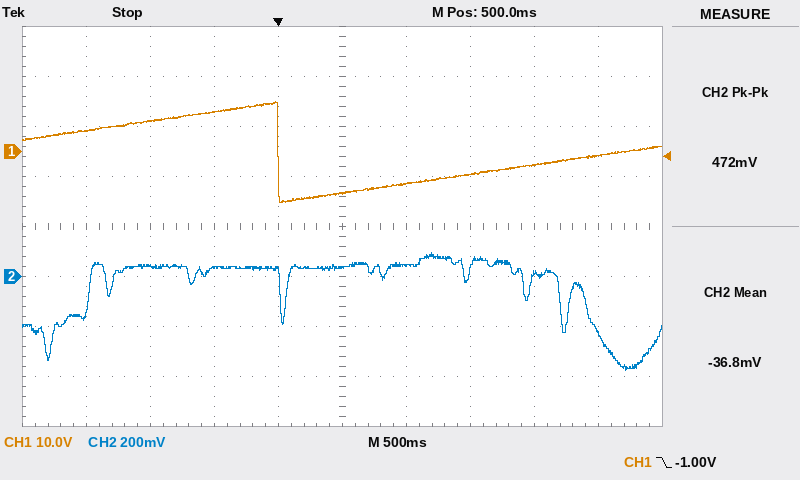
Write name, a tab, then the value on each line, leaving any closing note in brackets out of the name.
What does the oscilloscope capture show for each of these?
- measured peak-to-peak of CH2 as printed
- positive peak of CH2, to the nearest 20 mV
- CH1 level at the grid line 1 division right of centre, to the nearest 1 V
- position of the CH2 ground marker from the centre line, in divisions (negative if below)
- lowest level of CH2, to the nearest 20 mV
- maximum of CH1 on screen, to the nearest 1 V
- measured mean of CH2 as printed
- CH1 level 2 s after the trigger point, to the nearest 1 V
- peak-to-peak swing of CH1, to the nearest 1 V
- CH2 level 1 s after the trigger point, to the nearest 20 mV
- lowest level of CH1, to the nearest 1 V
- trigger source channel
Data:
measured peak-to-peak of CH2 as printed	472 mV
positive peak of CH2, to the nearest 20 mV	100 mV
CH1 level at the grid line 1 division right of centre, to the nearest 1 V	-6 V
position of the CH2 ground marker from the centre line, in divisions	-1.0 div
lowest level of CH2, to the nearest 20 mV	-380 mV
maximum of CH1 on screen, to the nearest 1 V	10 V
measured mean of CH2 as printed	-36.8 mV
CH1 level 2 s after the trigger point, to the nearest 1 V	-3 V
peak-to-peak swing of CH1, to the nearest 1 V	20 V
CH2 level 1 s after the trigger point, to the nearest 20 mV	40 mV
lowest level of CH1, to the nearest 1 V	-10 V
trigger source channel	CH1
